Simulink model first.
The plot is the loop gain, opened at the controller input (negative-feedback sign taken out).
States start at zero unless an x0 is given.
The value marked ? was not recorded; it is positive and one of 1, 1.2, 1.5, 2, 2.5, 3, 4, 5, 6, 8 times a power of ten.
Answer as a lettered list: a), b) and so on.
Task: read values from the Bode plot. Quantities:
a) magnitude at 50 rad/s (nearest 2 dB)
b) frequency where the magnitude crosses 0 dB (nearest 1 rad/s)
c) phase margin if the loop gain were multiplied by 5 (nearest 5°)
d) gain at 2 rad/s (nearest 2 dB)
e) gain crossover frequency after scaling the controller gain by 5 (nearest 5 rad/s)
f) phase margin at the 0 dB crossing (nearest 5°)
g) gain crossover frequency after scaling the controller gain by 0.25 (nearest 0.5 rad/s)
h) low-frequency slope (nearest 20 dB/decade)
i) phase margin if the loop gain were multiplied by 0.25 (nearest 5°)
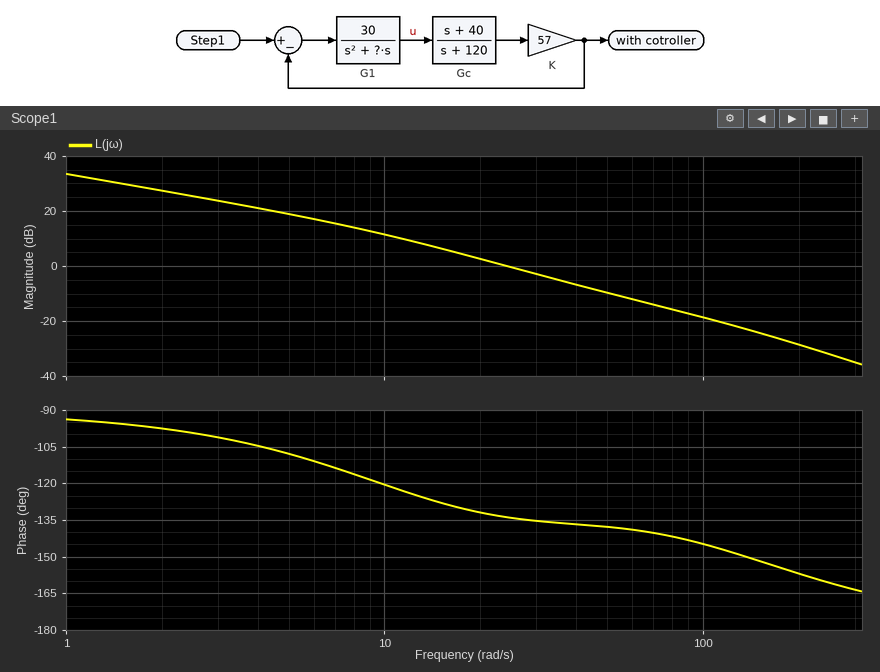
a) -10 dB
b) 24 rad/s
c) 40°
d) 28 dB
e) 70 rad/s
f) 45°
g) 9.5 rad/s
h) -20 dB/decade
i) 60°
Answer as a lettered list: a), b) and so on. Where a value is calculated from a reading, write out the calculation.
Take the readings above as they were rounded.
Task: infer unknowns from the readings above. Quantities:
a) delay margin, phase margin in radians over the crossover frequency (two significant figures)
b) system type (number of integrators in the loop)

a) 45 × π / 180 / 24 = 0.033 s
b) 1
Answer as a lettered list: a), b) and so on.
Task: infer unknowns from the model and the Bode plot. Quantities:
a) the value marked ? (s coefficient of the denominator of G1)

a) 12
